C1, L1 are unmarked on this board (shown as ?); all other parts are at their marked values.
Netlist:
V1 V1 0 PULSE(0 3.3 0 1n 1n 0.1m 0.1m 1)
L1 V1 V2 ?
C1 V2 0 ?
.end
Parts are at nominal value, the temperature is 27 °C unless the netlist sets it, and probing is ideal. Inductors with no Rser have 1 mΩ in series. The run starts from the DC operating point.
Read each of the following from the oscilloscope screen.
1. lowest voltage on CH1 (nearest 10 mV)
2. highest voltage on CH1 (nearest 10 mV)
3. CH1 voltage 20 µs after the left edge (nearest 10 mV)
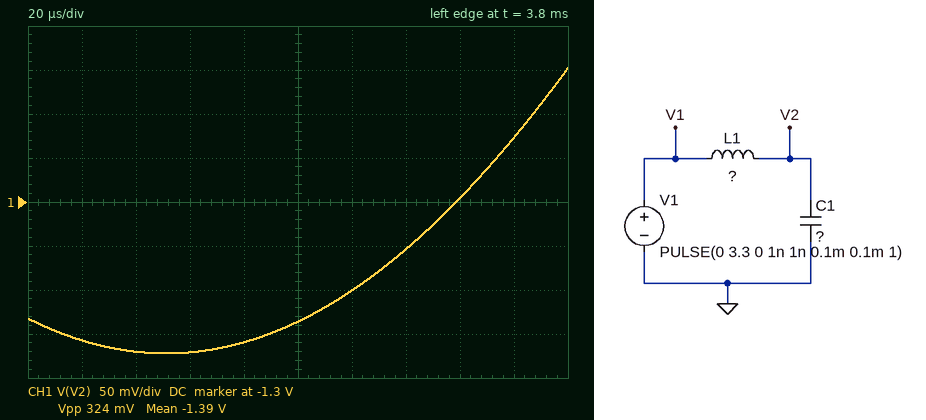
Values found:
-1.47 V
-1.15 V
-1.46 V
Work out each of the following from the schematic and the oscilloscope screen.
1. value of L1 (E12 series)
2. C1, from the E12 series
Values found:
220 µH
220 µF
